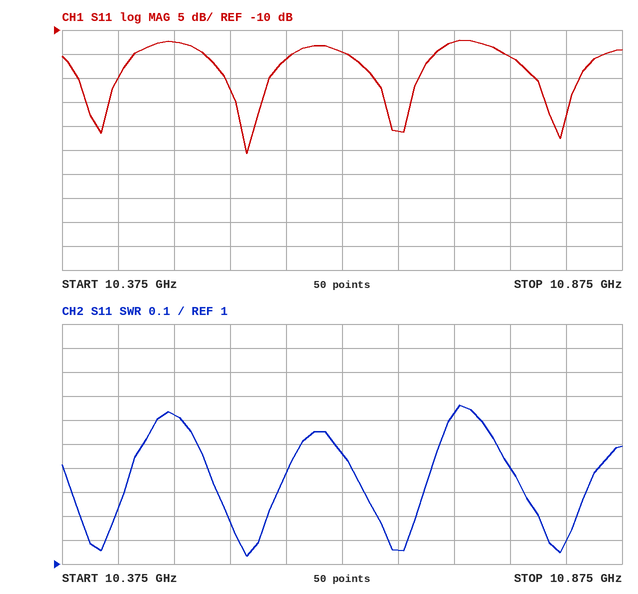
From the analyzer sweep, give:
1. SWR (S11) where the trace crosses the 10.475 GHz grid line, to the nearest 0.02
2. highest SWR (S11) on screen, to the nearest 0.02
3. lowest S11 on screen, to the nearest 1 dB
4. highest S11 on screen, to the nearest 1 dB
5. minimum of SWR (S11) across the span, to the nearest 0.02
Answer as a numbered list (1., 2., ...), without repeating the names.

1. 1.62
2. 1.66
3. -36 dB
4. -12 dB
5. 1.04
